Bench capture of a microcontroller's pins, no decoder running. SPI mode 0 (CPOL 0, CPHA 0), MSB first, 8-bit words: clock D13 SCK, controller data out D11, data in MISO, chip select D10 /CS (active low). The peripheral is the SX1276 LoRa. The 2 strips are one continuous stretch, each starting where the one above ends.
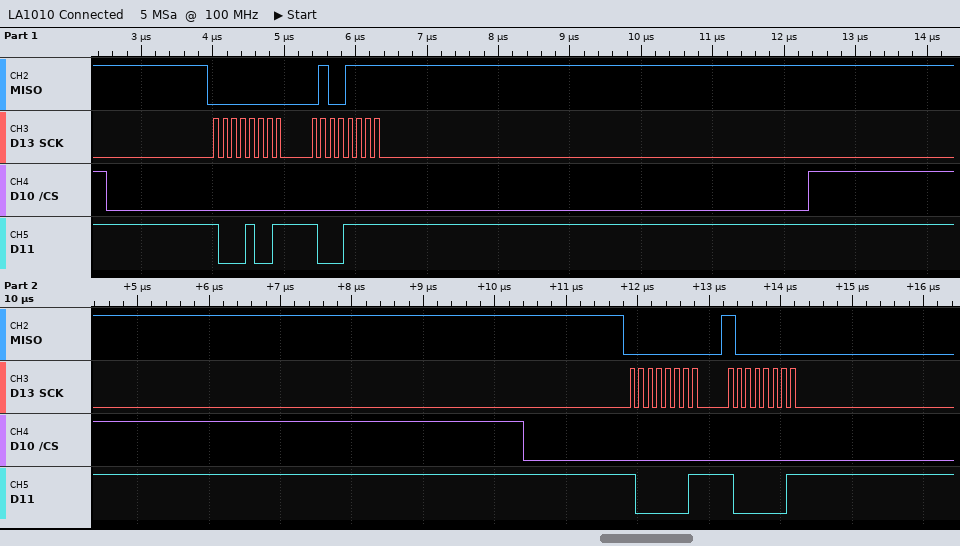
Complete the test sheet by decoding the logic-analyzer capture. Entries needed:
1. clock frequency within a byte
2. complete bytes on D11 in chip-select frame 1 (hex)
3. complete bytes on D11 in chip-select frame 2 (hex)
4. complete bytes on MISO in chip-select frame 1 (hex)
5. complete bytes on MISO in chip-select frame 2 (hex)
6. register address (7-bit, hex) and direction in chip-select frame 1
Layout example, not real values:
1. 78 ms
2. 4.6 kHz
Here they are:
1. 8 MHz
2. 0x89 0x8F
3. 0x81 0x81
4. 0x00 0x4F
5. 0x00 0x80
6. 0x09 write
